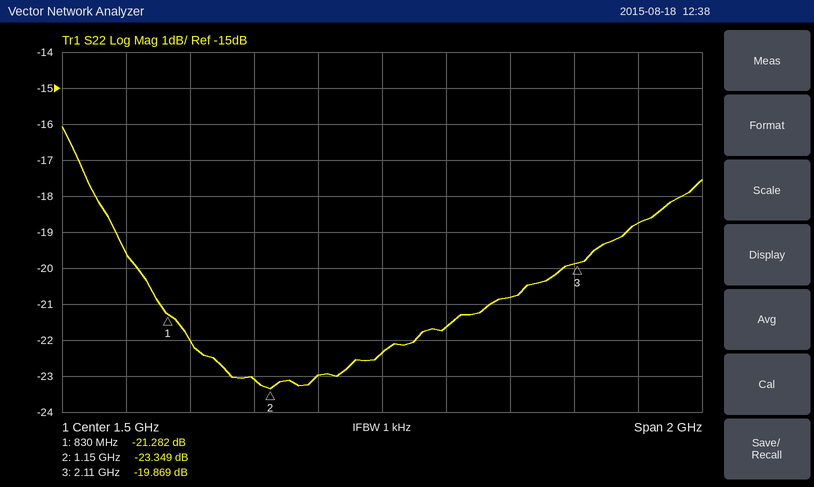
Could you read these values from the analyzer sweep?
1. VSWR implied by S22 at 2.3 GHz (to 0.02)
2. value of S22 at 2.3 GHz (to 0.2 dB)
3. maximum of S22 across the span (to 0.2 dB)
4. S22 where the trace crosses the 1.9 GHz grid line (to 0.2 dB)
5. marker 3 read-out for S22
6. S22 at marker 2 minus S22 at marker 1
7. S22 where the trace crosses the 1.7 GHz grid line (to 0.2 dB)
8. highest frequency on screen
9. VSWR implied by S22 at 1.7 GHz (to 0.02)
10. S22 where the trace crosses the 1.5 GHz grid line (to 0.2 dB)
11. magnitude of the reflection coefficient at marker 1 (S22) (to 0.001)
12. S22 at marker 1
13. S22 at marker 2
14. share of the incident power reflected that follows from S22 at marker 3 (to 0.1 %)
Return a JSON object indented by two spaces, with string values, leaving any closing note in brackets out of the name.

{
  "VSWR implied by S22 at 2.3 GHz": "1.26",
  "value of S22 at 2.3 GHz": "-18.8 dB",
  "maximum of S22 across the span": "-16.0 dB",
  "S22 where the trace crosses the 1.9 GHz grid line": "-20.8 dB",
  "marker 3 read-out for S22": "-19.869 dB",
  "S22 at marker 2 minus S22 at marker 1": "-2.067 dB",
  "S22 where the trace crosses the 1.7 GHz grid line": "-21.6 dB",
  "highest frequency on screen": "2.5 GHz",
  "VSWR implied by S22 at 1.7 GHz": "1.18",
  "S22 where the trace crosses the 1.5 GHz grid line": "-22.4 dB",
  "magnitude of the reflection coefficient at marker 1 (S22)": "0.086",
  "S22 at marker 1": "-21.282 dB",
  "S22 at marker 2": "-23.349 dB",
  "share of the incident power reflected that follows from S22 at marker 3": "1.0 %"
}
